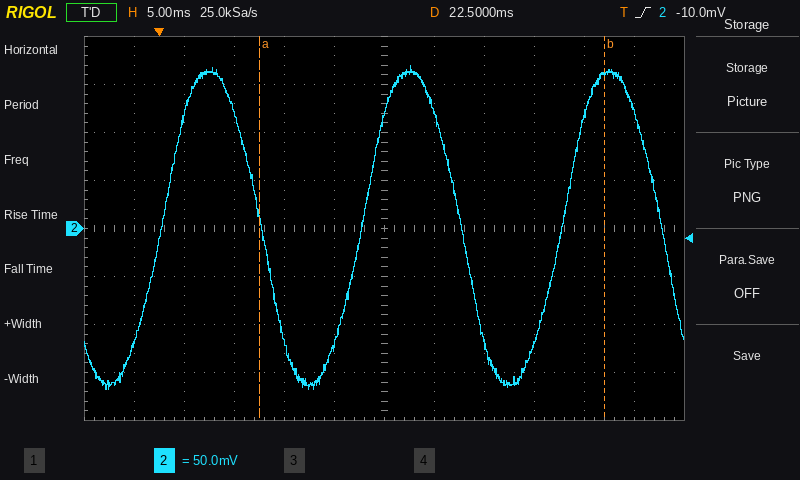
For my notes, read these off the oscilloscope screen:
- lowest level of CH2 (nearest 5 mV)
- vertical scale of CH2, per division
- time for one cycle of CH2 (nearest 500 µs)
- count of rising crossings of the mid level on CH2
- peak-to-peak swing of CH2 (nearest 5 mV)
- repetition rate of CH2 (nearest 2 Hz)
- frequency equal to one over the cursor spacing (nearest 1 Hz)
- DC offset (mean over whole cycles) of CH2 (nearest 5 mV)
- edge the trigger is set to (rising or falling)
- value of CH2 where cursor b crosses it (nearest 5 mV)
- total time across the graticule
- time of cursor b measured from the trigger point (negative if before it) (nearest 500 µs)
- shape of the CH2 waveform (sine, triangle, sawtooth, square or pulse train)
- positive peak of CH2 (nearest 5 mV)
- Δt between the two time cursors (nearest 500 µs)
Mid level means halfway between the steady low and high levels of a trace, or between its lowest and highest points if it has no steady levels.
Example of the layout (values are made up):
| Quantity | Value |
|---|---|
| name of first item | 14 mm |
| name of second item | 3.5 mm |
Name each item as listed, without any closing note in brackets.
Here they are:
| Quantity | Value |
|---|---|
| lowest level of CH2 | -170 mV |
| vertical scale of CH2, per division | 50 mV |
| time for one cycle of CH2 | 20.0 ms |
| count of rising crossings of the mid level on CH2 | 3 |
| peak-to-peak swing of CH2 | 340 mV |
| repetition rate of CH2 | 50 Hz |
| frequency equal to one over the cursor spacing | 29 Hz |
| DC offset (mean over whole cycles) of CH2 | 0 mV |
| edge the trigger is set to | rising |
| value of CH2 where cursor b crosses it | 160 mV |
| total time across the graticule | 60 ms |
| time of cursor b measured from the trigger point (negative if before it) | +44.5 ms |
| shape of the CH2 waveform | sine |
| positive peak of CH2 | 170 mV |
| Δt between the two time cursors | 34.5 ms |
